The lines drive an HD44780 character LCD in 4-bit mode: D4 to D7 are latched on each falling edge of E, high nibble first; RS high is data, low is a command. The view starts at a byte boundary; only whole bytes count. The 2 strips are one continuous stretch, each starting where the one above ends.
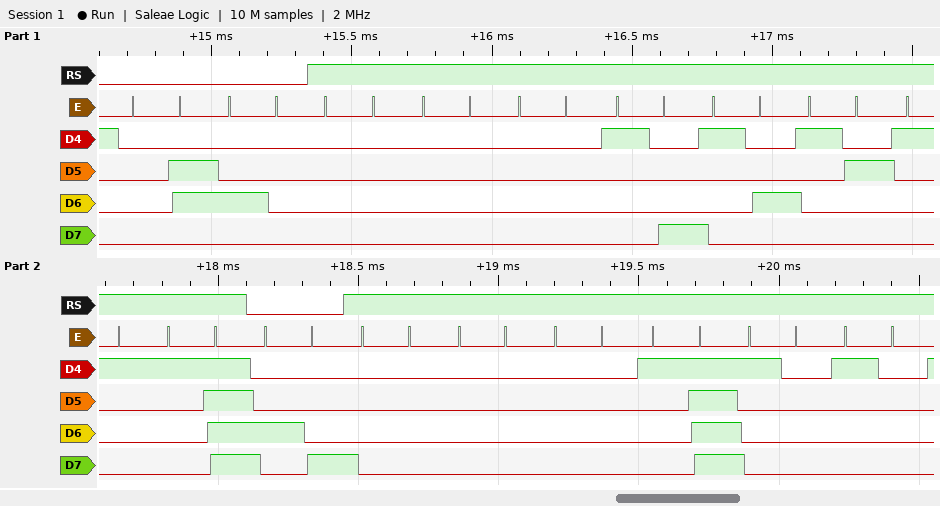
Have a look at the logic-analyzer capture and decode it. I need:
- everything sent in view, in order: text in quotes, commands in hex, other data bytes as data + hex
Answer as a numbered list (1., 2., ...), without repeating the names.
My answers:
1. 0x06 0x40 data 00 00 00 18 14 12 11 1F 0x48 data 00 00 00 1F 10 10
